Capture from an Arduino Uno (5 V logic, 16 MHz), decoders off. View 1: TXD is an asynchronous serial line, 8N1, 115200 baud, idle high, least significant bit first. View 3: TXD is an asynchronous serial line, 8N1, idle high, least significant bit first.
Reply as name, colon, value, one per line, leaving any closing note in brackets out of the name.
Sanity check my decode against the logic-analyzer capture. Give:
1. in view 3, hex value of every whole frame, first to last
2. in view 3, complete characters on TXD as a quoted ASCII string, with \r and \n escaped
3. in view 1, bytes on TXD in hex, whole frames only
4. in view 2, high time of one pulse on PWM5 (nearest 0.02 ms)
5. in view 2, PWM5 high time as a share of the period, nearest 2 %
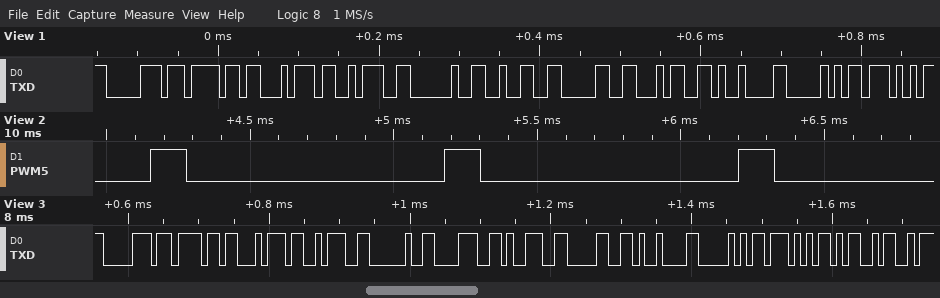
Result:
in view 3, hex value of every whole frame, first to last: 70 6F 74 3A 20 38 39 30 09 50 57 4D
in view 3, complete characters on TXD as a quoted ASCII string, with \r and \n escaped: "pot: 890\tPWM"
in view 1, bytes on TXD in hex, whole frames only: 70 6F 74 3A 20 32 30 34 09 50 57
in view 2, high time of one pulse on PWM5: 0.12 ms
in view 2, PWM5 high time as a share of the period, nearest 2 %: 12 %
